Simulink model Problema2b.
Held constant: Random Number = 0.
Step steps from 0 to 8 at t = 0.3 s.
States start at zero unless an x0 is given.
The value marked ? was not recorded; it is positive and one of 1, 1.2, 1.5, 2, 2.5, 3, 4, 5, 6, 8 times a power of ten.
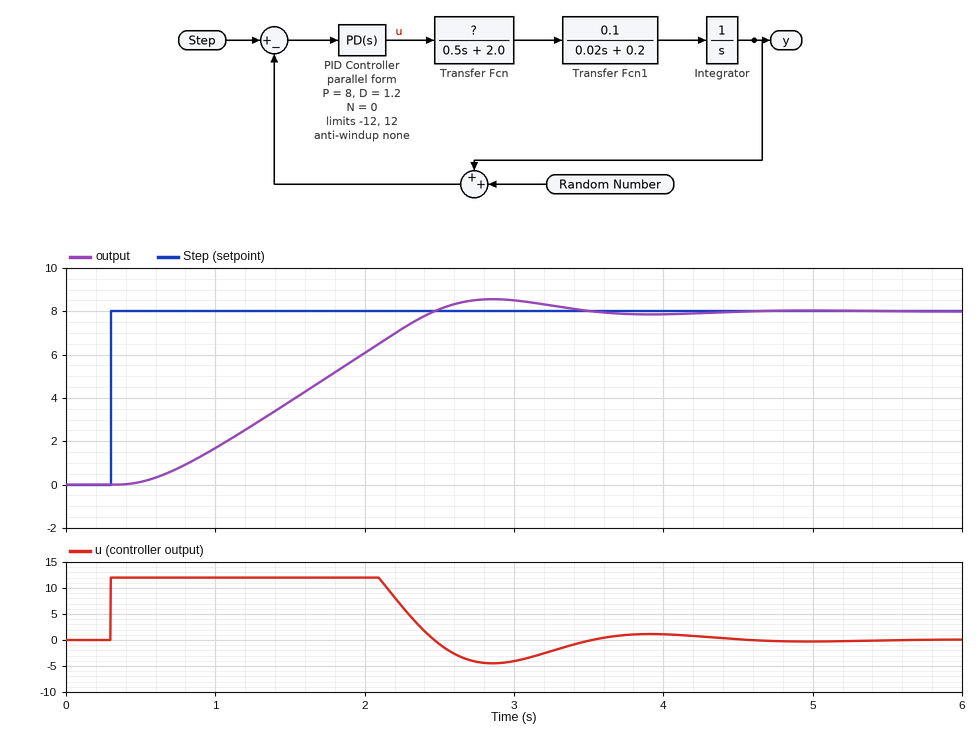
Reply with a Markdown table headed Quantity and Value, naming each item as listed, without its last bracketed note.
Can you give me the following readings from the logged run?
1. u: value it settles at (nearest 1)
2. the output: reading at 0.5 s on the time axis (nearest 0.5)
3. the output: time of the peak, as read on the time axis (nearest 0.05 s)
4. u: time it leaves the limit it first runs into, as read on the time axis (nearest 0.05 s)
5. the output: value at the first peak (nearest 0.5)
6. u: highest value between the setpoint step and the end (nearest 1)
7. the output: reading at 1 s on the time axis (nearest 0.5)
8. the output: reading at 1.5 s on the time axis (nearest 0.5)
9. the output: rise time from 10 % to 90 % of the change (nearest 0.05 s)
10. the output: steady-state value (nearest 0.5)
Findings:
| Quantity | Value |
|---|---|
| u: value it settles at | 0 |
| the output: reading at 0.5 s on the time axis | 0.0 |
| the output: time of the peak, as read on the time axis | 2.85 s |
| u: time it leaves the limit it first runs into, as read on the time axis | 2.10 s |
| the output: value at the first peak | 8.5 |
| u: highest value between the setpoint step and the end | 12 |
| the output: reading at 1 s on the time axis | 1.5 |
| the output: reading at 1.5 s on the time axis | 4.0 |
| the output: rise time from 10 % to 90 % of the change | 1.50 s |
| the output: steady-state value | 8.0 |
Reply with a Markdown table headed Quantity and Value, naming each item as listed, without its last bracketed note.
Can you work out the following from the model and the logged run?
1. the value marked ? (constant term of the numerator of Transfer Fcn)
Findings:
| Quantity | Value |
|---|---|
| the value marked ? | 1.5 |
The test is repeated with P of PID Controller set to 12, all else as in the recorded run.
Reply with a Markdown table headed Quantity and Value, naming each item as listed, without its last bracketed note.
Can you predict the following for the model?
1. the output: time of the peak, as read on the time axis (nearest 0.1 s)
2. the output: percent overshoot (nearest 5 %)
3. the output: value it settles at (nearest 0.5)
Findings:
| Quantity | Value |
|---|---|
| the output: time of the peak, as read on the time axis | 2.8 s |
| the output: percent overshoot | 10 % |
| the output: value it settles at | 8.0 |
